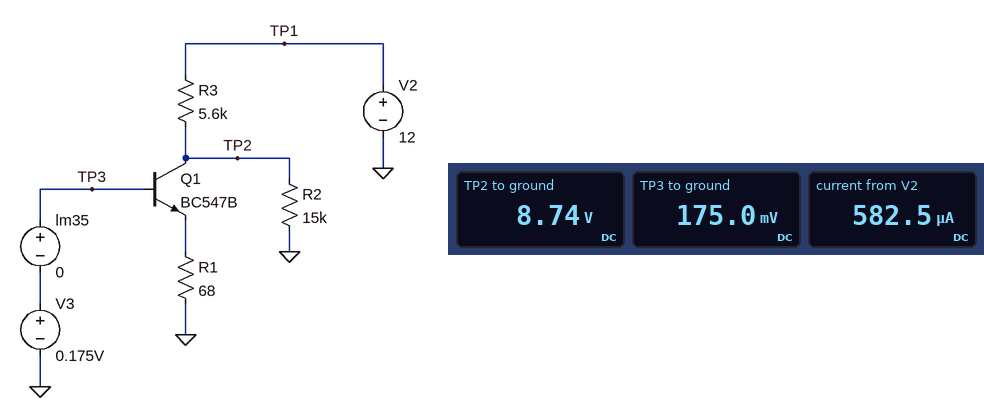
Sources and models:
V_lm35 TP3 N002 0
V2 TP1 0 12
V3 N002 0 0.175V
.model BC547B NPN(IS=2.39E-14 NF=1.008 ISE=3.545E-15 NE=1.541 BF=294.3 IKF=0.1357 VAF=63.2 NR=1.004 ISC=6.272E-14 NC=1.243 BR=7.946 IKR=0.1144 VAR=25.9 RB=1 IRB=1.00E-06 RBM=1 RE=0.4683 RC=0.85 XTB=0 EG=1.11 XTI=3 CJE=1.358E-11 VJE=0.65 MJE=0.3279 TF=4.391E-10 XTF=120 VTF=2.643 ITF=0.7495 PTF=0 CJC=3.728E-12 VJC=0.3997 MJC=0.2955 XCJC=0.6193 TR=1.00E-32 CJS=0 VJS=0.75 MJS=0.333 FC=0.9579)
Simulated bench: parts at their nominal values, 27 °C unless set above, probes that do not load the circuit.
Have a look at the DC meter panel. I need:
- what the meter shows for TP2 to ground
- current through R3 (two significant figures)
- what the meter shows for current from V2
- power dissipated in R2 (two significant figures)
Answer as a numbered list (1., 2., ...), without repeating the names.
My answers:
1. 8.74 V
2. 580 µA
3. 582.5 µA
4. 5.1 mW
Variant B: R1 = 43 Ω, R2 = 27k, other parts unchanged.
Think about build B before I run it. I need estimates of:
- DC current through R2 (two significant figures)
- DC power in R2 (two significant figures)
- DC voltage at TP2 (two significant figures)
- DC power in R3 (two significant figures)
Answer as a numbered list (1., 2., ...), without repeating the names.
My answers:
1. 370 µA
2. 3.7 mW
3. 9.9 V
4. 760 µW
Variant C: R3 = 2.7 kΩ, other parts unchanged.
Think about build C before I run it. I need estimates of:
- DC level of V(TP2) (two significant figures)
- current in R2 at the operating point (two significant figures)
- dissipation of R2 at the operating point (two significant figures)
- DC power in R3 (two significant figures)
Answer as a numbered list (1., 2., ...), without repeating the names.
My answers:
1. 10 V
2. 680 µA
3. 6.9 mW
4. 1.2 mW
